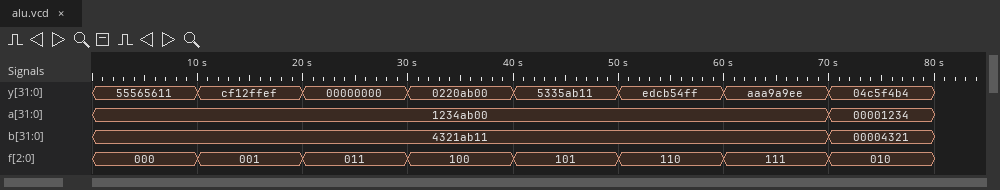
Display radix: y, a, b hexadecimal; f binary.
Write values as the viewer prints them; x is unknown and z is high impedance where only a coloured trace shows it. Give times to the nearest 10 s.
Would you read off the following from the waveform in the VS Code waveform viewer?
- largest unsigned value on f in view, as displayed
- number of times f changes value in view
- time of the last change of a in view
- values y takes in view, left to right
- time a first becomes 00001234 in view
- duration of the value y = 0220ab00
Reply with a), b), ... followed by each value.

a) 111
b) 7
c) 70 s
d) 55565611, cf12ffef, 00000000, 0220ab00, 5335ab11, edcb54ff, aaa9a9ee, 04c5f4b4
e) 70 s
f) 10 s
